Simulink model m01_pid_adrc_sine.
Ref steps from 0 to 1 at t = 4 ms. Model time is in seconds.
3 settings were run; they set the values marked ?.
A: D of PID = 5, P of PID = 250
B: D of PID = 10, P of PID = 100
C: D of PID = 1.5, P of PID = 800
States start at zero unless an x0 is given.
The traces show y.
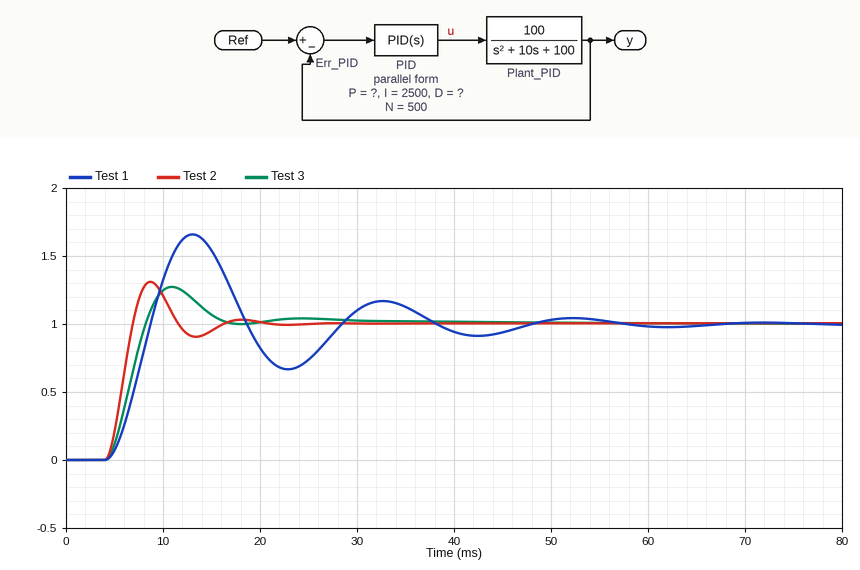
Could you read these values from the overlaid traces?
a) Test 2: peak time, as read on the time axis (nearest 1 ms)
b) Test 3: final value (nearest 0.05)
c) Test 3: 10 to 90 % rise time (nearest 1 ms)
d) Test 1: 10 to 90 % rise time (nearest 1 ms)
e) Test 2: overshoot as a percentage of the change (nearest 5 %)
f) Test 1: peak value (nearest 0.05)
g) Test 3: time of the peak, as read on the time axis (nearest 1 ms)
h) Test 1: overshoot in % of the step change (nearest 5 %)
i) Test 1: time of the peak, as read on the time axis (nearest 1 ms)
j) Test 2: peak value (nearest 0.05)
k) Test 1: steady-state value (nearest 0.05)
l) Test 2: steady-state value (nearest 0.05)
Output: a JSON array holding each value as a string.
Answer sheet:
["9 ms", "1.00", "3 ms", "3 ms", "30 %", "1.65", "11 ms", "65 %", "13 ms", "1.30", "1.00", "1.00"]
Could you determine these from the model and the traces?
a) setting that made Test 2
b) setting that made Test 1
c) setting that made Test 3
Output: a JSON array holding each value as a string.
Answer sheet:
["B", "C", "A"]
